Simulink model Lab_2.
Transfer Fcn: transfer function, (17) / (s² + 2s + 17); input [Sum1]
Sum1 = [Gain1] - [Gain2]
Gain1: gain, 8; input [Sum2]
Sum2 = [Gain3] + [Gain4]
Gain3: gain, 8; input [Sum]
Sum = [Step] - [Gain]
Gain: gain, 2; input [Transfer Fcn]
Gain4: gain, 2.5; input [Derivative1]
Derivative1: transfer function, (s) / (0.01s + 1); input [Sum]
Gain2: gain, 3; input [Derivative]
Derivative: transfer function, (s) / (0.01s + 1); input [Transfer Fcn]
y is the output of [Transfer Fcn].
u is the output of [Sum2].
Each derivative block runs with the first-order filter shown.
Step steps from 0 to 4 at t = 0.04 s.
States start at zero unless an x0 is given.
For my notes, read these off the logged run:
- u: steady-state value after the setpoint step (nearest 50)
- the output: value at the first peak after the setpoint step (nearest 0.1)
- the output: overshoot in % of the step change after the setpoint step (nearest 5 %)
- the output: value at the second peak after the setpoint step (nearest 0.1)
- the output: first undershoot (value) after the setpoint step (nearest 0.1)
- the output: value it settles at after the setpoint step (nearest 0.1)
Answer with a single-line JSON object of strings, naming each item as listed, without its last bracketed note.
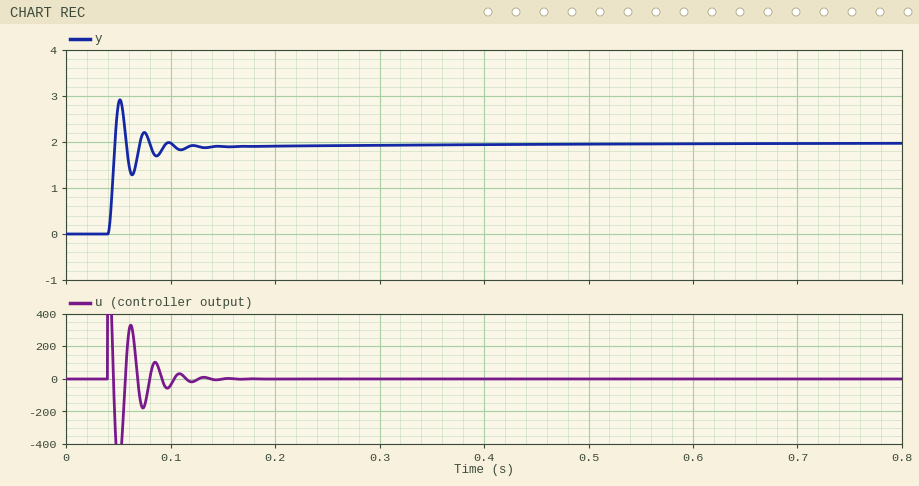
{"u: steady-state value after the setpoint step": "0", "the output: value at the first peak after the setpoint step": "2.9", "the output: overshoot in % of the step change after the setpoint step": "45 %", "the output: value at the second peak after the setpoint step": "2.2", "the output: first undershoot (value) after the setpoint step": "1.3", "the output: value it settles at after the setpoint step": "2.0"}
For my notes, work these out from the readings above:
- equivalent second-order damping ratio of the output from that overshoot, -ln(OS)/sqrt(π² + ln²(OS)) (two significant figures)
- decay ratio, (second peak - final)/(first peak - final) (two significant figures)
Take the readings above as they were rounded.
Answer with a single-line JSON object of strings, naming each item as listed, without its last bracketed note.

{"equivalent second-order damping ratio of the output from that overshoot, -ln(OS)/sqrt(π² + ln²(OS))": "0.25", "decay ratio, (second peak - final)/(first peak - final)": "0.22"}
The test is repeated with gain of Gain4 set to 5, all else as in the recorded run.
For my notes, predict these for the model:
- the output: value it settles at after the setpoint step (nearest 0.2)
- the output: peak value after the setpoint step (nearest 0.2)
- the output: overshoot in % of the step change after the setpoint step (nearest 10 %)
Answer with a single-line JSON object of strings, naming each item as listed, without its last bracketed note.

{"the output: value it settles at after the setpoint step": "2.0", "the output: peak value after the setpoint step": "3.2", "the output: overshoot in % of the step change after the setpoint step": "60 %"}
